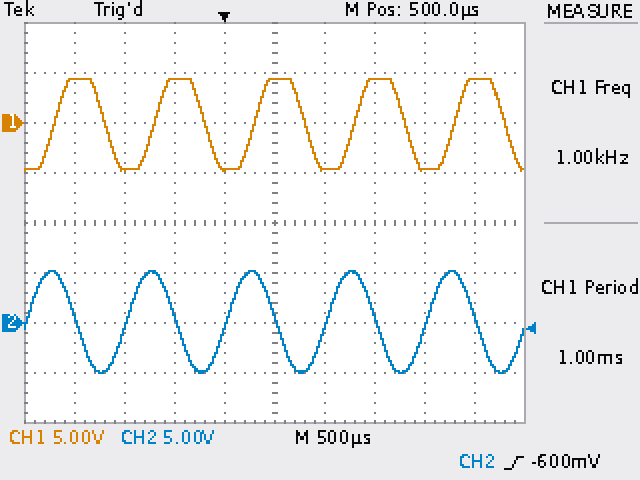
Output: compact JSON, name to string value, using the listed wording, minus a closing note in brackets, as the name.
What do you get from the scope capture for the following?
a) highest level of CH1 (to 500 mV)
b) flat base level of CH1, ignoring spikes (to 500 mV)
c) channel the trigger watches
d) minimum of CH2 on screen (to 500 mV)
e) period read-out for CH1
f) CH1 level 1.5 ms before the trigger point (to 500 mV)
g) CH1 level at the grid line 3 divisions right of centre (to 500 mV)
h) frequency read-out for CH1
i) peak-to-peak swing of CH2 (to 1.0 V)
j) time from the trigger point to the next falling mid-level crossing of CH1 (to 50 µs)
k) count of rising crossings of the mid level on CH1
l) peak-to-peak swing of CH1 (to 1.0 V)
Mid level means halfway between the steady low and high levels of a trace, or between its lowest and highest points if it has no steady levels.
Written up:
{"highest level of CH1": "4.5 V", "flat base level of CH1, ignoring spikes": "-4.5 V", "channel the trigger watches": "CH2", "minimum of CH2 on screen": "-5.0 V", "period read-out for CH1": "1.00 ms", "CH1 level 1.5 ms before the trigger point": "4.5 V", "CH1 level at the grid line 3 divisions right of centre": "-4.5 V", "frequency read-out for CH1": "1.00 kHz", "peak-to-peak swing of CH2": "10.0 V", "time from the trigger point to the next falling mid-level crossing of CH1": "800 µs", "count of rising crossings of the mid level on CH1": "5", "peak-to-peak swing of CH1": "9.0 V"}
